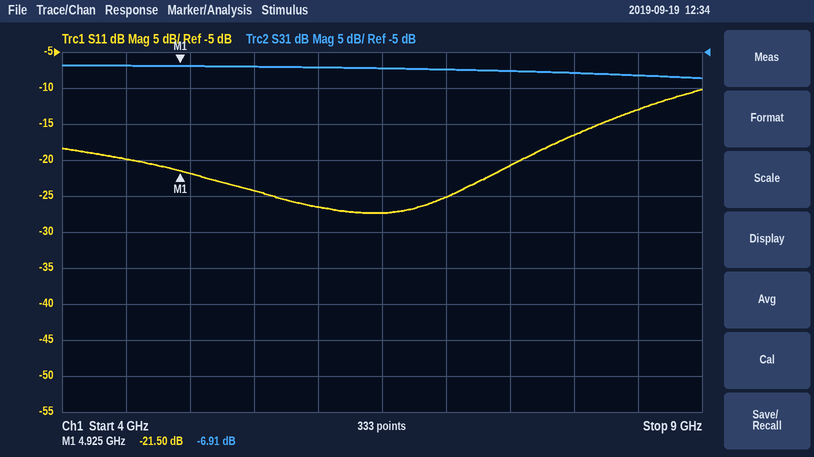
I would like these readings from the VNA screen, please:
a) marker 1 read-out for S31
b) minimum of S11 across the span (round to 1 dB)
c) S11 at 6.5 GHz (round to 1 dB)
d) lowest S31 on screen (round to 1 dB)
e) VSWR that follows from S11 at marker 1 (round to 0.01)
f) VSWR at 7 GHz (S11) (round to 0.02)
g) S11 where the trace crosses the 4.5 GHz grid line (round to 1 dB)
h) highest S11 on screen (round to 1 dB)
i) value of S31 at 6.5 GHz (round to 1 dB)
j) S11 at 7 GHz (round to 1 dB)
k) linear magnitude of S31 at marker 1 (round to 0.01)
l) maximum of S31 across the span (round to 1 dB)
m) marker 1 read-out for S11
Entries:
-6.91 dB
-27 dB
-27 dB
-9 dB
1.18
1.12
-20 dB
-10 dB
-7 dB
-25 dB
0.45
-7 dB
-21.50 dB
